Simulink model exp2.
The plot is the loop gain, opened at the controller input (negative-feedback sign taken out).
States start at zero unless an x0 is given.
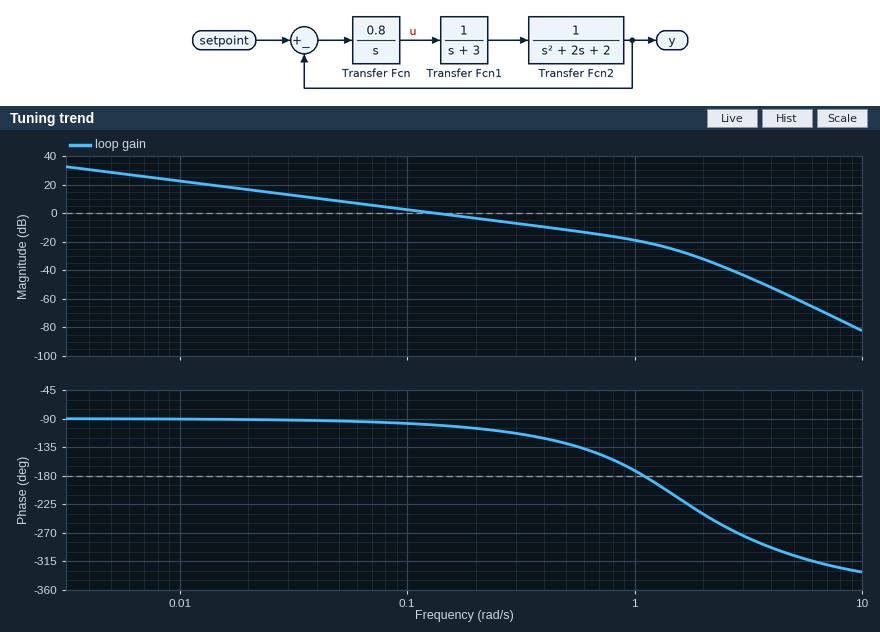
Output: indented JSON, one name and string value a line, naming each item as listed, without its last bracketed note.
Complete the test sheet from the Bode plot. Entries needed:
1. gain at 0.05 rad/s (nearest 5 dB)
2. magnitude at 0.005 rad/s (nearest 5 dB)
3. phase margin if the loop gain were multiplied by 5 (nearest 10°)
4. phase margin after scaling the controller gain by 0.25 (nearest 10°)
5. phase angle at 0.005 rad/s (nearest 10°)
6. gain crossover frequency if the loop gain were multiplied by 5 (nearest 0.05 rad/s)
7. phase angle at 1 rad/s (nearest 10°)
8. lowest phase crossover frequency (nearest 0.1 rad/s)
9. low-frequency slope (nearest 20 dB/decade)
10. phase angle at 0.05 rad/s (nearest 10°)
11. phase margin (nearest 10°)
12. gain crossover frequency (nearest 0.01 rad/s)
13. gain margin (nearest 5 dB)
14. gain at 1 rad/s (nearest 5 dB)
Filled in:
{
  "gain at 0.05 rad/s": "10 dB",
  "magnitude at 0.005 rad/s": "30 dB",
  "phase margin if the loop gain were multiplied by 5": "40°",
  "phase margin after scaling the controller gain by 0.25": "90°",
  "phase angle at 0.005 rad/s": "-90°",
  "gain crossover frequency if the loop gain were multiplied by 5": "0.65 rad/s",
  "phase angle at 1 rad/s": "-170°",
  "lowest phase crossover frequency": "1.1 rad/s",
  "low-frequency slope": "-20 dB/decade",
  "phase angle at 0.05 rad/s": "-90°",
  "phase margin": "80°",
  "gain crossover frequency": "0.13 rad/s",
  "gain margin": "20 dB",
  "gain at 1 rad/s": "-20 dB"
}
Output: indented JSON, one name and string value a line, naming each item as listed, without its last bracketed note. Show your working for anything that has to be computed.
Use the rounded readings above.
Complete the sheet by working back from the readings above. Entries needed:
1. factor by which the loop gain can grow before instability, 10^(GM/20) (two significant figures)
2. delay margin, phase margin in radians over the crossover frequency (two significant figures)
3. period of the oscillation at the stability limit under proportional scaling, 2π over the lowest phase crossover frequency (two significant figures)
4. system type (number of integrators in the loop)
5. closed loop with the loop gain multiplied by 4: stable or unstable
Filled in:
{
  "factor by which the loop gain can grow before instability, 10^(GM/20)": "10^(20 / 20) = 10",
  "delay margin, phase margin in radians over the crossover frequency": "80 × π / 180 / 0.13 = 11 s",
  "period of the oscillation at the stability limit under proportional scaling, 2π over the lowest phase crossover frequency": "2π / 1.1 = 5.7 s",
  "system type": "1",
  "closed loop with the loop gain multiplied by 4: stable or unstable": "stable"
}
